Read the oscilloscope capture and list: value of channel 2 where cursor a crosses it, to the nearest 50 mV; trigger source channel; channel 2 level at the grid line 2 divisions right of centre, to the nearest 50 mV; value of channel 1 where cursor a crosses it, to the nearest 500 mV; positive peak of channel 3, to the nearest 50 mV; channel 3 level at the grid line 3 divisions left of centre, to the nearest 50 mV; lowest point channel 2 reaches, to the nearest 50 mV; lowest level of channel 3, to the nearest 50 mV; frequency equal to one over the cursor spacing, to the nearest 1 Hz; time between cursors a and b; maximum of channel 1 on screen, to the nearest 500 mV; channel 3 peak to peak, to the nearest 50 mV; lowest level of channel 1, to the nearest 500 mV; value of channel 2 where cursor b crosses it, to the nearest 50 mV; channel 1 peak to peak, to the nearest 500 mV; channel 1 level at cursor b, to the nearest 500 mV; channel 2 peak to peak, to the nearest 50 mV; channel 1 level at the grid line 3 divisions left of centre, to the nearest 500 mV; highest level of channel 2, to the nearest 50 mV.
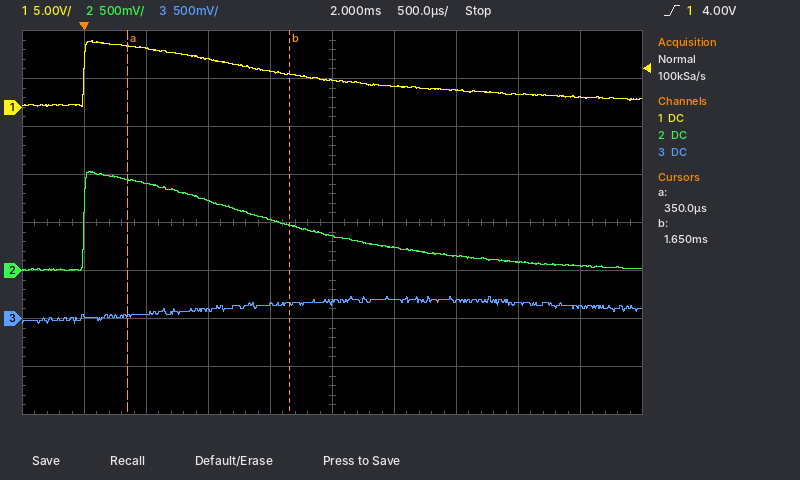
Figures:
950 mV
channel 1
150 mV
6.5 V
250 mV
50 mV
0 mV
-50 mV
769 Hz
1.30 ms
7.0 V
300 mV
0.0 V
450 mV
7.0 V
3.5 V
1.05 V
6.0 V
1.05 V
